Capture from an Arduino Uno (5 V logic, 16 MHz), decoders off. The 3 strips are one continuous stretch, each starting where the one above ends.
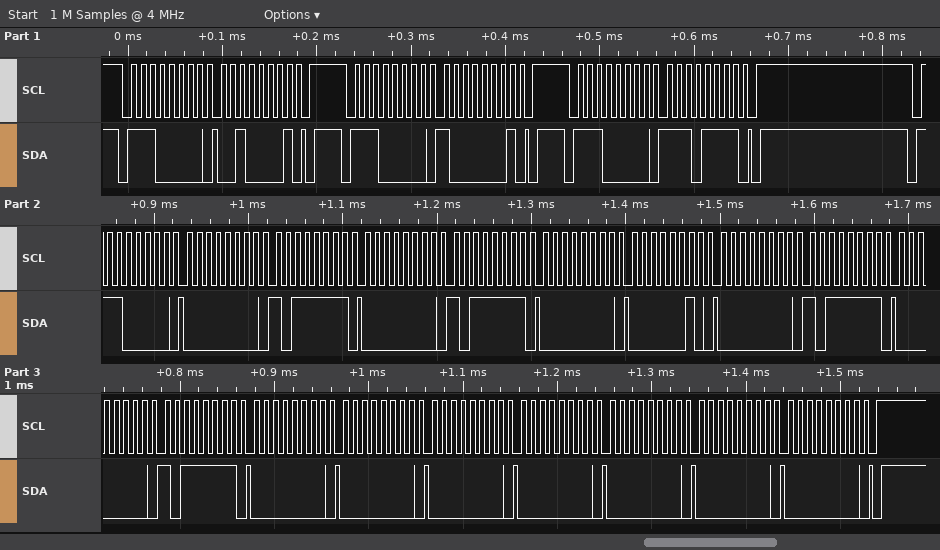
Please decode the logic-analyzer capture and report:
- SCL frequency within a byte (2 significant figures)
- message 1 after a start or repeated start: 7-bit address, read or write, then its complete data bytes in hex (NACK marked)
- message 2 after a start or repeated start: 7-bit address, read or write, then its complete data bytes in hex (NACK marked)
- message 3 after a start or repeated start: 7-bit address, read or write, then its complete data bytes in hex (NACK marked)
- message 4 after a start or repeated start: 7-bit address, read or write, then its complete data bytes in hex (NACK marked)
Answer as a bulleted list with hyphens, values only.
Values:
- 100 kHz
- 0x70 write: 21
- 0x70 write: 81
- 0x70 write: EF
- 0x70 write: 00 BF 00 BF 00 02 00 BF 00 BF 00 00 00 00 00 00 00
